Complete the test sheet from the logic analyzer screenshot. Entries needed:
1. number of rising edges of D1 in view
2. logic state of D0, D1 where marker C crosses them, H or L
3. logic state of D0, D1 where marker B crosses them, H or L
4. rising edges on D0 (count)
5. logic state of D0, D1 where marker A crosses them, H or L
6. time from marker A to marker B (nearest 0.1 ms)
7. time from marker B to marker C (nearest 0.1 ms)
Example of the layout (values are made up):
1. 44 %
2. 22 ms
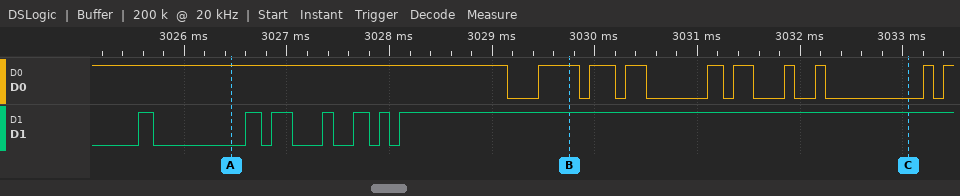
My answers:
1. 7
2. D0=L, D1=H
3. D0=H, D1=H
4. 9
5. D0=H, D1=L
6. 3.3 ms
7. 3.3 ms
